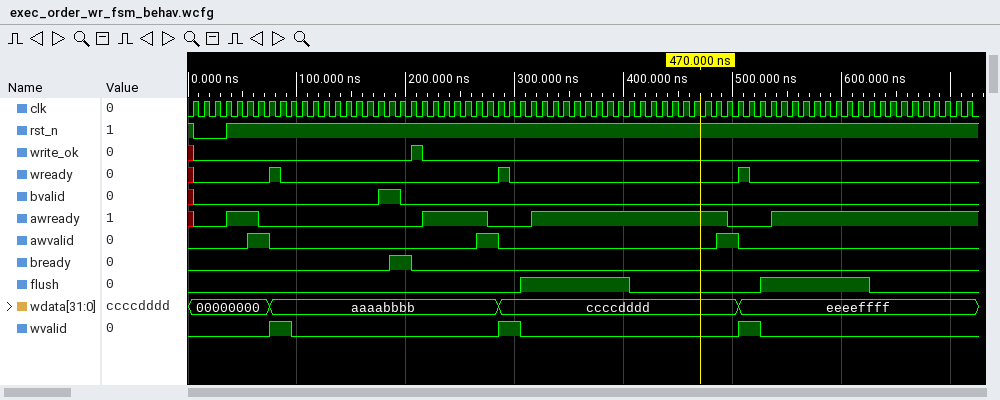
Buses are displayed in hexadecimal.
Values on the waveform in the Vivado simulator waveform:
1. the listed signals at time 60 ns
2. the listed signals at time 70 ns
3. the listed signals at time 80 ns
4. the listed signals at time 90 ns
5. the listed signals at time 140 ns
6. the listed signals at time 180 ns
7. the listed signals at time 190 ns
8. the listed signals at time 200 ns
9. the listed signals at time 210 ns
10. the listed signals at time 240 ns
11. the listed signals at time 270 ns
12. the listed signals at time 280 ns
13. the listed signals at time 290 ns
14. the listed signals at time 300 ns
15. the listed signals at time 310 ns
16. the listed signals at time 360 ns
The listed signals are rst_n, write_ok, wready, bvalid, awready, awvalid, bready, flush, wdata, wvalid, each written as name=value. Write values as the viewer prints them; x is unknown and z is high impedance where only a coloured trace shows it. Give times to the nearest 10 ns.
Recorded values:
rst_n=1, write_ok=0, wready=0, bvalid=0, awready=1, awvalid=1, bready=0, flush=0, wdata=00000000, wvalid=0
rst_n=1, write_ok=0, wready=0, bvalid=0, awready=0, awvalid=1, bready=0, flush=0, wdata=00000000, wvalid=0
rst_n=1, write_ok=0, wready=1, bvalid=0, awready=0, awvalid=0, bready=0, flush=0, wdata=aaaabbbb, wvalid=1
rst_n=1, write_ok=0, wready=0, bvalid=0, awready=0, awvalid=0, bready=0, flush=0, wdata=aaaabbbb, wvalid=1
rst_n=1, write_ok=0, wready=0, bvalid=0, awready=0, awvalid=0, bready=0, flush=0, wdata=aaaabbbb, wvalid=0
rst_n=1, write_ok=0, wready=0, bvalid=1, awready=0, awvalid=0, bready=0, flush=0, wdata=aaaabbbb, wvalid=0
rst_n=1, write_ok=0, wready=0, bvalid=1, awready=0, awvalid=0, bready=1, flush=0, wdata=aaaabbbb, wvalid=0
rst_n=1, write_ok=0, wready=0, bvalid=0, awready=0, awvalid=0, bready=1, flush=0, wdata=aaaabbbb, wvalid=0
rst_n=1, write_ok=1, wready=0, bvalid=0, awready=0, awvalid=0, bready=0, flush=0, wdata=aaaabbbb, wvalid=0
rst_n=1, write_ok=0, wready=0, bvalid=0, awready=1, awvalid=0, bready=0, flush=0, wdata=aaaabbbb, wvalid=0
rst_n=1, write_ok=0, wready=0, bvalid=0, awready=1, awvalid=1, bready=0, flush=0, wdata=aaaabbbb, wvalid=0
rst_n=1, write_ok=0, wready=0, bvalid=0, awready=0, awvalid=1, bready=0, flush=0, wdata=aaaabbbb, wvalid=0
rst_n=1, write_ok=0, wready=1, bvalid=0, awready=0, awvalid=0, bready=0, flush=0, wdata=ccccdddd, wvalid=1
rst_n=1, write_ok=0, wready=0, bvalid=0, awready=0, awvalid=0, bready=0, flush=0, wdata=ccccdddd, wvalid=1
rst_n=1, write_ok=0, wready=0, bvalid=0, awready=0, awvalid=0, bready=0, flush=1, wdata=ccccdddd, wvalid=0
rst_n=1, write_ok=0, wready=0, bvalid=0, awready=1, awvalid=0, bready=0, flush=1, wdata=ccccdddd, wvalid=0
